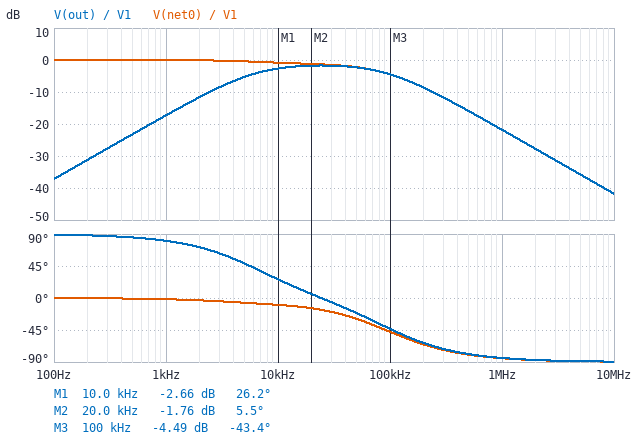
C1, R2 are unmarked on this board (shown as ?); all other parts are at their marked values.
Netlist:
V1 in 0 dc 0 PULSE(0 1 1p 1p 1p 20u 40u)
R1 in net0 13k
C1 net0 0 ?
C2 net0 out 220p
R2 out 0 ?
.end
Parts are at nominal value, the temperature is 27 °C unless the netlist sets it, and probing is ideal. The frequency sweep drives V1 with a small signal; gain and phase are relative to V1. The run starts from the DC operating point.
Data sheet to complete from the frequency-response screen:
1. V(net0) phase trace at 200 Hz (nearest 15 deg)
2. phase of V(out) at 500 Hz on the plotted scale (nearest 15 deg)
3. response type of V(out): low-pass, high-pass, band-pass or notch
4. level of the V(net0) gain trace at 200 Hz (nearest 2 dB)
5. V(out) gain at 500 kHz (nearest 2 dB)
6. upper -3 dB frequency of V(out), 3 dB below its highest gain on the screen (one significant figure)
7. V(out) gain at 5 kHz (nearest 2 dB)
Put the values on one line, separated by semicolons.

0 deg; 90 deg; band-pass; 0 dB; -16 dB; 100 kHz; -6 dB
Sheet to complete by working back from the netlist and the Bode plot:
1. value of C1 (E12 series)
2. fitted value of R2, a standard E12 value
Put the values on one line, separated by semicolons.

150 pF; 100 kΩ
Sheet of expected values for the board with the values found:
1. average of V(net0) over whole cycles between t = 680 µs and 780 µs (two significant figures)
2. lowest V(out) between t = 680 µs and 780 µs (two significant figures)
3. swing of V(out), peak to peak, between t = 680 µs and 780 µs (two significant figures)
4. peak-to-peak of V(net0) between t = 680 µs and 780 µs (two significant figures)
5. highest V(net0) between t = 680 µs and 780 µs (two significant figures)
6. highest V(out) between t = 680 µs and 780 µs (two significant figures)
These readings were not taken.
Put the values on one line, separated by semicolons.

500 mV; -480 mV; 970 mV; 920 mV; 960 mV; 480 mV
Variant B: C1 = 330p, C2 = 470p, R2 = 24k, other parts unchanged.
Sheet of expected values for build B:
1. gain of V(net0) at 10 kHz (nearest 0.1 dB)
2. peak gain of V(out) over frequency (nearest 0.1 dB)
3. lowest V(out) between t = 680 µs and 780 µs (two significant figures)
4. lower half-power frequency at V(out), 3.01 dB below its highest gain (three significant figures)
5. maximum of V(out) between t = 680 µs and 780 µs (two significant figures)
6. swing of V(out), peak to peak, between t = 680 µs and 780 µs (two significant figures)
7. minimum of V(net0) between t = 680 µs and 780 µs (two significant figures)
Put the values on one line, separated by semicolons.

-2.2 dB; -5.7 dB; -310 mV; 6.71 kHz; 310 mV; 610 mV; 120 mV
